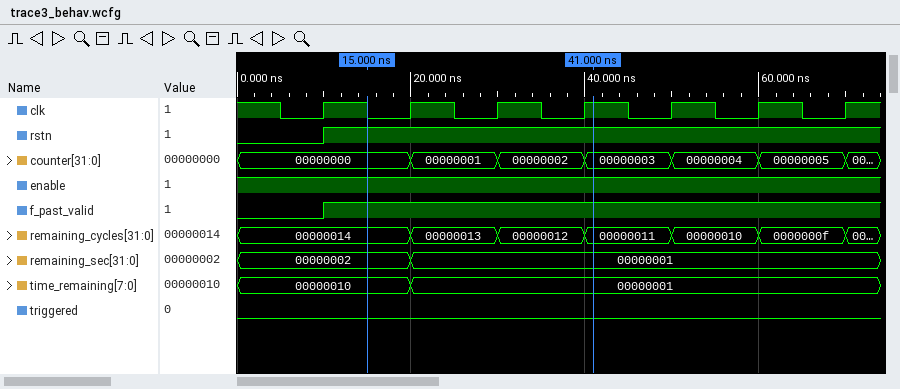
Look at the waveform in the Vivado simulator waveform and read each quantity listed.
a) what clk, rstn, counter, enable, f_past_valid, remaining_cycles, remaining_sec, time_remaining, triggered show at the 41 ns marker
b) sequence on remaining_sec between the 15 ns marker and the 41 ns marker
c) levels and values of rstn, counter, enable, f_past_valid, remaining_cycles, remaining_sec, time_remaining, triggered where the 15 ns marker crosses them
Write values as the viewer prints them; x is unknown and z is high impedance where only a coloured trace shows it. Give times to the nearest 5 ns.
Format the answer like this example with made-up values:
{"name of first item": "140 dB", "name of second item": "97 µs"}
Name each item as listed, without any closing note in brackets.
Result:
{"what clk, rstn, counter, enable, f_past_valid, remaining_cycles, remaining_sec, time_remaining, triggered show at the 41 ns marker": "clk=1, rstn=1, counter=00000003, enable=1, f_past_valid=1, remaining_cycles=00000011, remaining_sec=00000001, time_remaining=00000001, triggered=0", "sequence on remaining_sec between the 15 ns marker and the 41 ns marker": "00000002, 00000001", "levels and values of rstn, counter, enable, f_past_valid, remaining_cycles, remaining_sec, time_remaining, triggered where the 15 ns marker crosses them": "rstn=1, counter=00000000, enable=1, f_past_valid=1, remaining_cycles=00000014, remaining_sec=00000002, time_remaining=00000010, triggered=0"}
